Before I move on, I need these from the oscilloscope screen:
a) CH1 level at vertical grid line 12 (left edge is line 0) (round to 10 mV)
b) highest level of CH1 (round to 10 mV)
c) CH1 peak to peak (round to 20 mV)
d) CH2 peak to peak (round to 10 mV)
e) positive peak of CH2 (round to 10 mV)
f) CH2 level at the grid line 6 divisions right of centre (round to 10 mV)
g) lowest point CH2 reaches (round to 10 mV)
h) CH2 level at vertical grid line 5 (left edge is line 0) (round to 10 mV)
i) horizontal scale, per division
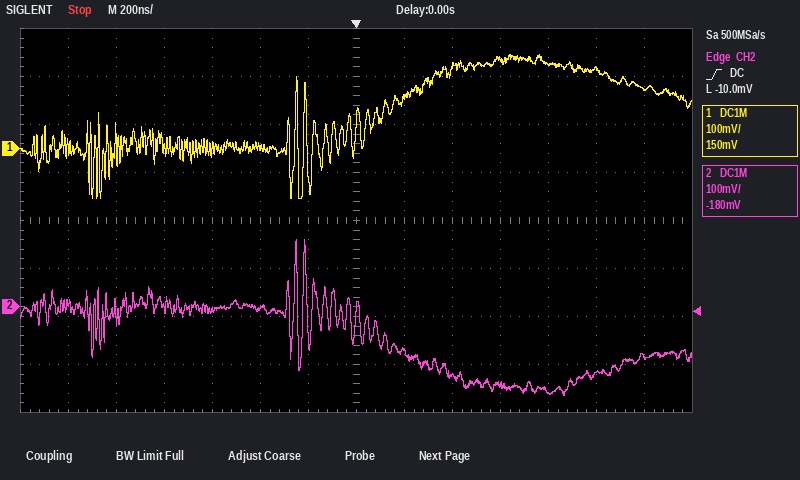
170 mV
200 mV
300 mV
320 mV
140 mV
-100 mV
-180 mV
0 mV
200 ns
